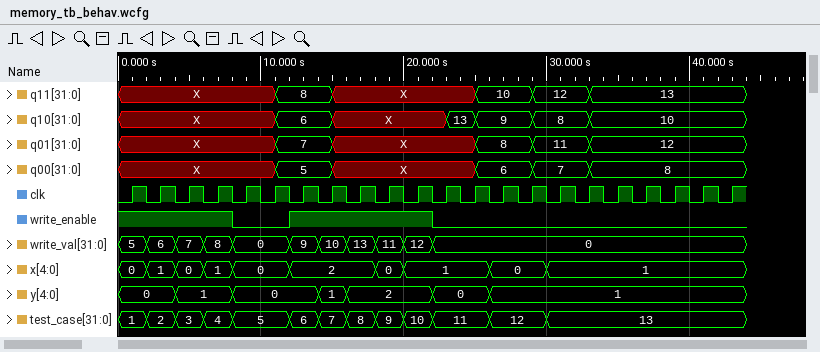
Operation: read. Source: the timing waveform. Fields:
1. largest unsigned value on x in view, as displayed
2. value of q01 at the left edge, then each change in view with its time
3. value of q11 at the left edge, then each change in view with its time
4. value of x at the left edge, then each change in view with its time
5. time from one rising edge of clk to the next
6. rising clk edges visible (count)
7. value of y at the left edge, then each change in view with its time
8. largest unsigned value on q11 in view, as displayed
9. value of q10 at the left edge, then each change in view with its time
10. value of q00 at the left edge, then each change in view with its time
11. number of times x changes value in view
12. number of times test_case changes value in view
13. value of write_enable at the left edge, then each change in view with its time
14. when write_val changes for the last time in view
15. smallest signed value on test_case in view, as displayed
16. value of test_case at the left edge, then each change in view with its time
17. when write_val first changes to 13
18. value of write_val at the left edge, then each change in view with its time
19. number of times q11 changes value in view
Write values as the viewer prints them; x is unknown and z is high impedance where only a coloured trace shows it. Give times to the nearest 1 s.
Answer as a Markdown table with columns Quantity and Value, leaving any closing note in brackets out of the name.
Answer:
| Quantity | Value |
|---|---|
| largest unsigned value on x in view, as displayed | 2 |
| value of q01 at the left edge, then each change in view with its time | X, 7 at 11 s, X at 15 s, 8 at 25 s, 11 at 29 s, 12 at 33 s |
| value of q11 at the left edge, then each change in view with its time | X, 8 at 11 s, X at 15 s, 10 at 25 s, 12 at 29 s, 13 at 33 s |
| value of x at the left edge, then each change in view with its time | 0, 1 at 2 s, 0 at 4 s, 1 at 6 s, 0 at 8 s, 2 at 12 s, 0 at 18 s, 1 at 20 s, 0 at 26 s, 1 at 30 s |
| time from one rising edge of clk to the next | 2 s |
| rising clk edges visible | 22 |
| value of y at the left edge, then each change in view with its time | 0, 1 at 4 s, 0 at 8 s, 1 at 14 s, 2 at 16 s, 0 at 22 s, 1 at 26 s |
| largest unsigned value on q11 in view, as displayed | 13 |
| value of q10 at the left edge, then each change in view with its time | X, 6 at 11 s, X at 15 s, 13 at 23 s, 9 at 25 s, 8 at 29 s, 10 at 33 s |
| value of q00 at the left edge, then each change in view with its time | X, 5 at 11 s, X at 15 s, 6 at 25 s, 7 at 29 s, 8 at 33 s |
| number of times x changes value in view | 9 |
| number of times test_case changes value in view | 12 |
| value of write_enable at the left edge, then each change in view with its time | 1, 0 at 8 s, 1 at 12 s, 0 at 22 s |
| when write_val changes for the last time in view | 22 s |
| smallest signed value on test_case in view, as displayed | 1 |
| value of test_case at the left edge, then each change in view with its time | 1, 2 at 2 s, 3 at 4 s, 4 at 6 s, 5 at 8 s, 6 at 12 s, 7 at 14 s, 8 at 16 s, 9 at 18 s, 10 at 20 s, 11 at 22 s, 12 at 26 s, 13 at 30 s |
| when write_val first changes to 13 | 16 s |
| value of write_val at the left edge, then each change in view with its time | 5, 6 at 2 s, 7 at 4 s, 8 at 6 s, 0 at 8 s, 9 at 12 s, 10 at 14 s, 13 at 16 s, 11 at 18 s, 12 at 20 s, 0 at 22 s |
| number of times q11 changes value in view | 5 |
